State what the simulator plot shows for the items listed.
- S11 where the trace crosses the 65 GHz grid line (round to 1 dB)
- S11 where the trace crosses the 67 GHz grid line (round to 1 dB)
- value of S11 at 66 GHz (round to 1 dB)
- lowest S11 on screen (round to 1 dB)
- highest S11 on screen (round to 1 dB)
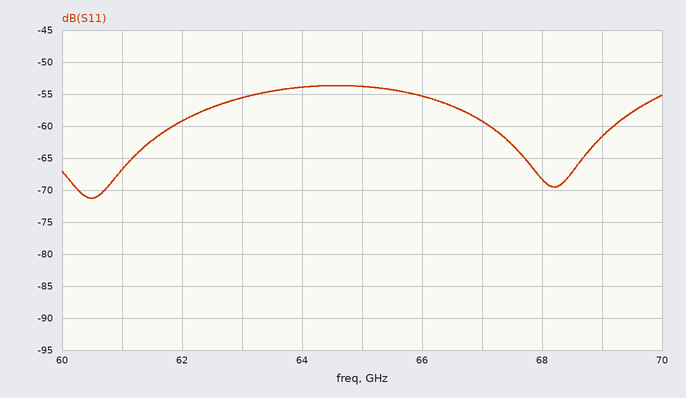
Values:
-54 dB
-59 dB
-55 dB
-71 dB
-54 dB
